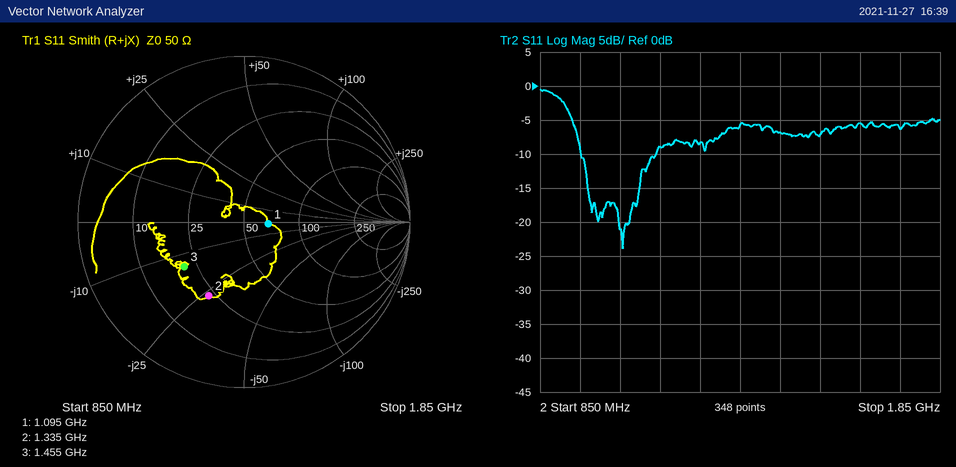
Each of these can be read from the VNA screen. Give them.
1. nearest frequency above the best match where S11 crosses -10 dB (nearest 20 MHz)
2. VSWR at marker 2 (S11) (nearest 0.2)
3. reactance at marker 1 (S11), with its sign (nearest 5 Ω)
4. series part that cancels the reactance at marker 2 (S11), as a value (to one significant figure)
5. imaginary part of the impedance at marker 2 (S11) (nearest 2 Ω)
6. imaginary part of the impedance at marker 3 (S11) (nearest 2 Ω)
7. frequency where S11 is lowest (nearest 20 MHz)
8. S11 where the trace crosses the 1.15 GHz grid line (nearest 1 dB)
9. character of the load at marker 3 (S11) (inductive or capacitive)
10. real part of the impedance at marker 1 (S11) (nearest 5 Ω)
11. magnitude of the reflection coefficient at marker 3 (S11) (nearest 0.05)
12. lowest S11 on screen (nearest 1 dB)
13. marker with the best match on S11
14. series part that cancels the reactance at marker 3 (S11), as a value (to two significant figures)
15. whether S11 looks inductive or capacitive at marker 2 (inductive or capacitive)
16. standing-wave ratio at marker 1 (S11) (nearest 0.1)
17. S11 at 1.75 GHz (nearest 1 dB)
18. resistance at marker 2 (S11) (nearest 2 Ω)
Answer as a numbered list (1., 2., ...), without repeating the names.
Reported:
1. 1.14 GHz
2. 3.0
3. 0 Ω
4. 3 nH
5. -26 Ω
6. -14 Ω
7. 1.06 GHz
8. -9 dB
9. capacitive
10. 65 Ω
11. 0.45
12. -24 dB
13. marker 1
14. 1.5 nH
15. capacitive
16. 1.3
17. -6 dB
18. 22 Ω
